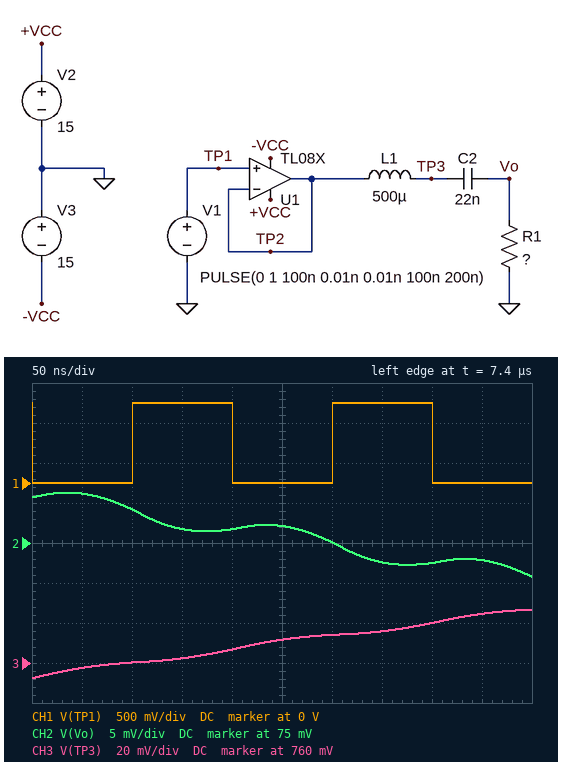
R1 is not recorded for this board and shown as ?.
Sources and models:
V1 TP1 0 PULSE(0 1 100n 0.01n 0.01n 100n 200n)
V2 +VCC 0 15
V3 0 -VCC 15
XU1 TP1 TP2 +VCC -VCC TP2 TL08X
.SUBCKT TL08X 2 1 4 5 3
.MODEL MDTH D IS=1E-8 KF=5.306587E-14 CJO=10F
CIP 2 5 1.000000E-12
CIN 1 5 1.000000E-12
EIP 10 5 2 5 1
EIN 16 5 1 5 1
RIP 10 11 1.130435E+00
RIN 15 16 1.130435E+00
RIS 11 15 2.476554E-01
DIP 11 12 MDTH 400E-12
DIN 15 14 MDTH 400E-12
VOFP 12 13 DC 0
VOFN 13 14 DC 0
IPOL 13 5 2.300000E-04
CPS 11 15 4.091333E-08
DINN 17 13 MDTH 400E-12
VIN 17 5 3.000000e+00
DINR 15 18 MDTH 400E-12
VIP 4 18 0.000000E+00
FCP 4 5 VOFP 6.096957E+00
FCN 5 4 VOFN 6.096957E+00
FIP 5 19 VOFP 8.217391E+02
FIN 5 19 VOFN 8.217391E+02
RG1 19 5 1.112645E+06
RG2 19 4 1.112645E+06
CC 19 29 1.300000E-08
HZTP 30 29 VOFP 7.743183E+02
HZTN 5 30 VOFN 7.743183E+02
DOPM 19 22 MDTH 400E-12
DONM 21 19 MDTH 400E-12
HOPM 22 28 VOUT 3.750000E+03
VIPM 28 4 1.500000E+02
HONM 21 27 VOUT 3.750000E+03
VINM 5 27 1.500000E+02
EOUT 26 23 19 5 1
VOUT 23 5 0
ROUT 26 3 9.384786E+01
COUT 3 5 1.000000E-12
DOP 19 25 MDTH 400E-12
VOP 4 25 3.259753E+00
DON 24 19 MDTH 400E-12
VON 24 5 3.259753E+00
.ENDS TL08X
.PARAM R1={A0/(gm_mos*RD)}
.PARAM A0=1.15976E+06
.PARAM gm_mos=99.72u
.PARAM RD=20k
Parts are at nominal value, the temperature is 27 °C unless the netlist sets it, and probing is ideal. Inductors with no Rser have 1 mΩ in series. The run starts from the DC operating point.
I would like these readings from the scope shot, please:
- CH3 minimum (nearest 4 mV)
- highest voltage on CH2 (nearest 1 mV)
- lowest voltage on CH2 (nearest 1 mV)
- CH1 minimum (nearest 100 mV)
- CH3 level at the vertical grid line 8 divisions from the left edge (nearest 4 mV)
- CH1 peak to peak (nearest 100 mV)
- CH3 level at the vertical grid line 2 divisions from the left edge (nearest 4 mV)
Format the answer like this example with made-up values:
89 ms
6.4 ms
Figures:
752 mV
81 mV
71 mV
0 V
780 mV
1.0 V
760 mV
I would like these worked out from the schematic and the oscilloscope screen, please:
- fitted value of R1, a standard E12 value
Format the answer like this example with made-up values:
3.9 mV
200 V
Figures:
39 Ω
